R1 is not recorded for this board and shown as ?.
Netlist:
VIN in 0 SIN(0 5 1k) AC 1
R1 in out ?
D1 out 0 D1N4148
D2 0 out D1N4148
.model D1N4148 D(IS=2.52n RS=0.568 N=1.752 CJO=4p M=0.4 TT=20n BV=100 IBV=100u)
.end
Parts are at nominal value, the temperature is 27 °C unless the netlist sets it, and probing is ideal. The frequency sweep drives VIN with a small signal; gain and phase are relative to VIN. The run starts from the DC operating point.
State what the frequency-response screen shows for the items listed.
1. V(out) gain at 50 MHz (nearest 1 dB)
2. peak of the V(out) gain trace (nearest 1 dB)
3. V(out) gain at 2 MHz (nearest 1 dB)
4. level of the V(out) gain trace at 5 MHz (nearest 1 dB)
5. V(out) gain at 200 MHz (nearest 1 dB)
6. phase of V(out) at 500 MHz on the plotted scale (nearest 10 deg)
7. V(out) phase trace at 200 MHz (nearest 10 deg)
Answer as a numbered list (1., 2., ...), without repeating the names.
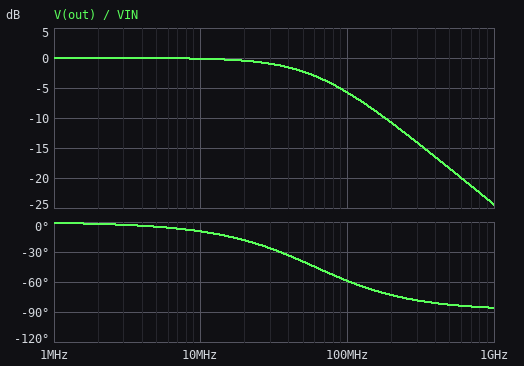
1. -2 dB
2. 0 dB
3. 0 dB
4. 0 dB
5. -11 dB
6. -80 deg
7. -70 deg
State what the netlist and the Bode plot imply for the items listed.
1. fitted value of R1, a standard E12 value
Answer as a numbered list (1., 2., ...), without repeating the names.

1. 330 Ω
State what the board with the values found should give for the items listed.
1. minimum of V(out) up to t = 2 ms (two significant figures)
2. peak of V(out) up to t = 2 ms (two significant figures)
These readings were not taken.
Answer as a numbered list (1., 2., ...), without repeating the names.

1. -710 mV
2. 710 mV
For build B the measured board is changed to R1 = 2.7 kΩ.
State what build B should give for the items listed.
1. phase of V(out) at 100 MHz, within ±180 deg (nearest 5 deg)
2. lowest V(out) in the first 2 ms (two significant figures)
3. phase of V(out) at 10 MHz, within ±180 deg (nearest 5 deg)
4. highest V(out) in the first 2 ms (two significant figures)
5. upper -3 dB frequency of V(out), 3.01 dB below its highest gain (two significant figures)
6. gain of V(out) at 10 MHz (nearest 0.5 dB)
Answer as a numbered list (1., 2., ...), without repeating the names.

1. -85 deg
2. -610 mV
3. -55 deg
4. 610 mV
5. 7.4 MHz
6. -4.5 dB
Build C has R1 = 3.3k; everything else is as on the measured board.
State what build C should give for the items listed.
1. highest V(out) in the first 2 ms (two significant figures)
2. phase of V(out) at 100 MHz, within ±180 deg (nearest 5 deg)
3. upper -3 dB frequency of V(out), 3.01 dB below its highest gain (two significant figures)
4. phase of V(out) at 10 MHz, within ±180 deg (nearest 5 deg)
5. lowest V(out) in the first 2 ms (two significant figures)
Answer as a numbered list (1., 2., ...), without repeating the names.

1. 600 mV
2. -85 deg
3. 6.0 MHz
4. -60 deg
5. -600 mV
